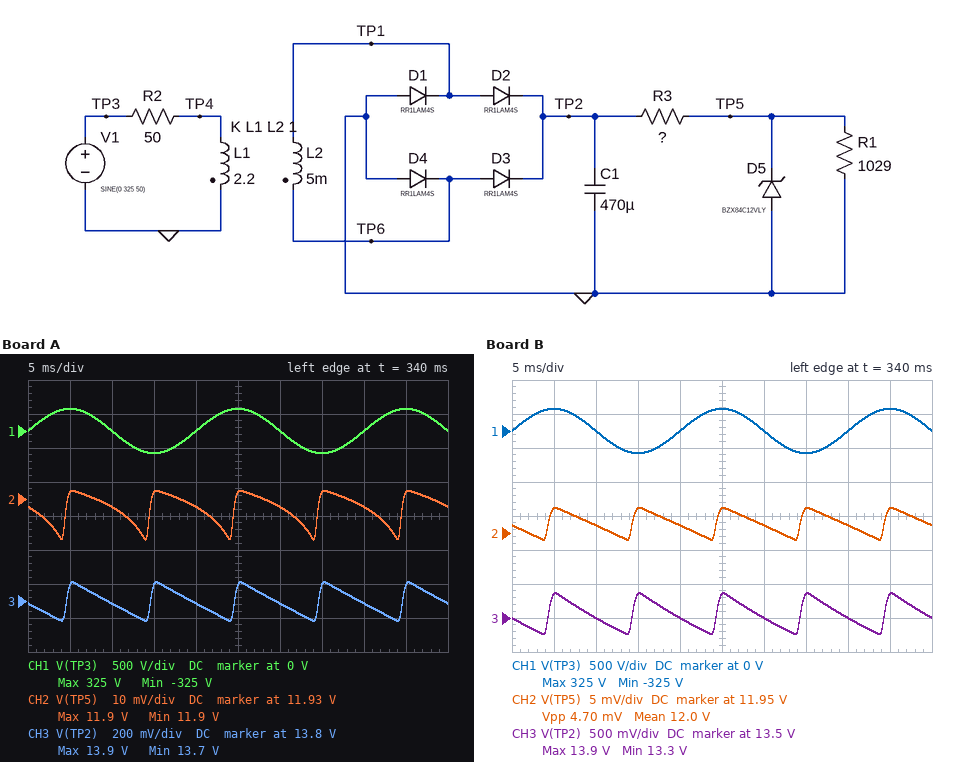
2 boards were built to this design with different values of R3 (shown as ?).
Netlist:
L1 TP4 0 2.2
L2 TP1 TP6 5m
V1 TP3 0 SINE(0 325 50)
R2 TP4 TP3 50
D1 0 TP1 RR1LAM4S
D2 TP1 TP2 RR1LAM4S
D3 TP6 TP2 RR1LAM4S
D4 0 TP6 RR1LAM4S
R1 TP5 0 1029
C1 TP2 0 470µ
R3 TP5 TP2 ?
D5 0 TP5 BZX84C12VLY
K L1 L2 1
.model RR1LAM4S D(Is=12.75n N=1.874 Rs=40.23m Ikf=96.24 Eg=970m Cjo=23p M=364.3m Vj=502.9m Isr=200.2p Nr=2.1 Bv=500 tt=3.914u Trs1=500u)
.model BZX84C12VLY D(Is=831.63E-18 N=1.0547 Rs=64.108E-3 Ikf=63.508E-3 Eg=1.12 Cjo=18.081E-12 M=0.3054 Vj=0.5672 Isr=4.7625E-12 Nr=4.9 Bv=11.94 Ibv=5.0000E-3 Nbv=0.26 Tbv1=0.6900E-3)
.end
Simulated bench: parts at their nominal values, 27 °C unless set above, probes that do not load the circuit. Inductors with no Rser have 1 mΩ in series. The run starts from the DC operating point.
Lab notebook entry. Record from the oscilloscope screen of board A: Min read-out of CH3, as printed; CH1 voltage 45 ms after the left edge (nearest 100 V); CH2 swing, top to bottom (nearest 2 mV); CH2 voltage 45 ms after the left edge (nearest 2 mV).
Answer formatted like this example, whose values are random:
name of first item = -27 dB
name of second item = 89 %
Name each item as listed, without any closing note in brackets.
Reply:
Min read-out of CH3, as printed = 13.7 V
CH1 voltage 45 ms after the left edge = 300 V
CH2 swing, top to bottom = 14 mV
CH2 voltage 45 ms after the left edge = 11.932 V
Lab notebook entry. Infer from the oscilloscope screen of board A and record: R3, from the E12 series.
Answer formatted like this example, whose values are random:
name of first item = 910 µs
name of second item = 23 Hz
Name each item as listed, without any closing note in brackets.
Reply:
R3, from the E12 series = 150 Ω
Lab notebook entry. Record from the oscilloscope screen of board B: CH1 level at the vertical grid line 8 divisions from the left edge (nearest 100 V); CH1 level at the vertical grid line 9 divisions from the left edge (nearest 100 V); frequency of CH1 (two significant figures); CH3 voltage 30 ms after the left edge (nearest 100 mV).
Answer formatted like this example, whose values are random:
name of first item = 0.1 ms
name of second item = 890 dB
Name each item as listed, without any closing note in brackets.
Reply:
CH1 level at the vertical grid line 8 divisions from the left edge = 0 V
CH1 level at the vertical grid line 9 divisions from the left edge = 300 V
frequency of CH1 = 50 Hz
CH3 voltage 30 ms after the left edge = 13.5 V
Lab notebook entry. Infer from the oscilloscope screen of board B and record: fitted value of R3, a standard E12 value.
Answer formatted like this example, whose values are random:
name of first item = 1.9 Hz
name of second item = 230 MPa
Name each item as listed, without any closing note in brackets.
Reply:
fitted value of R3, a standard E12 value = 47 Ω
